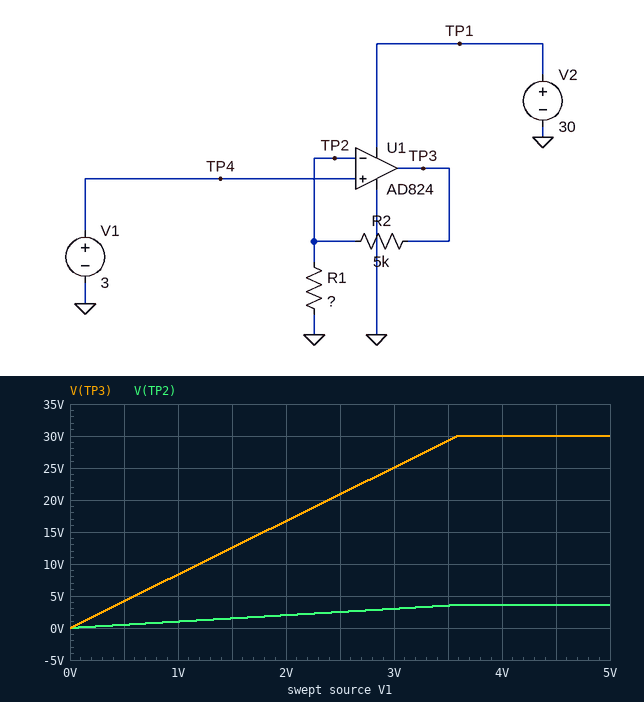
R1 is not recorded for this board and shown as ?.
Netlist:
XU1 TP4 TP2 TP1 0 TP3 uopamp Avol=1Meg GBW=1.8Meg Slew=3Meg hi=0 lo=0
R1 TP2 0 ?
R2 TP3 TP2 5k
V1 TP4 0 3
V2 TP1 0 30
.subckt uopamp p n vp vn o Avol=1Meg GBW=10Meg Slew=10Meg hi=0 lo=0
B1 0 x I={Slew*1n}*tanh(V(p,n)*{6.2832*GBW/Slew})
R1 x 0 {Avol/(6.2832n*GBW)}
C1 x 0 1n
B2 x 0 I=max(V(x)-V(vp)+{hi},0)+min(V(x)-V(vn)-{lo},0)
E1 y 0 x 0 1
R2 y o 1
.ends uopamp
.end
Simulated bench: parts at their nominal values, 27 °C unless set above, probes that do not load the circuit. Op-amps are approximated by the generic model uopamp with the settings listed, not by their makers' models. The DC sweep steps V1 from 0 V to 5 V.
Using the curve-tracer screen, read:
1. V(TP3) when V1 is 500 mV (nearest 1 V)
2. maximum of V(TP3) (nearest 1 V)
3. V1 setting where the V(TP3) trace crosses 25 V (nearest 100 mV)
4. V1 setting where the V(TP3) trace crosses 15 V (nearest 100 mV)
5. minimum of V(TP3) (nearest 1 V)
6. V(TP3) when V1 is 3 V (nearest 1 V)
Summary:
4 V
30 V
3.0 V
1.8 V
0 V
25 V
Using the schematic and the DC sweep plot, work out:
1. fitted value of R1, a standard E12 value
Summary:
680 Ω
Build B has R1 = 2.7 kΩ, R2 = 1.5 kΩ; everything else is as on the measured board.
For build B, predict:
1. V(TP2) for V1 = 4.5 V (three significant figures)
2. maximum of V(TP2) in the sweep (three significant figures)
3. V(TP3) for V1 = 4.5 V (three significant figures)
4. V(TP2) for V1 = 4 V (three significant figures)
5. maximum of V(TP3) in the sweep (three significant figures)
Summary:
4.50 V
5.00 V
7.00 V
4.00 V
7.78 V
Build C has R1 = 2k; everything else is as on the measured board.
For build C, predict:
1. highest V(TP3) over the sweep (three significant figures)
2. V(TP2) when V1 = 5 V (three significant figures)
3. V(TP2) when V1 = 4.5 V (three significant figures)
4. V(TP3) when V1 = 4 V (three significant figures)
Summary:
17.5 V
5.00 V
4.50 V
14.0 V
